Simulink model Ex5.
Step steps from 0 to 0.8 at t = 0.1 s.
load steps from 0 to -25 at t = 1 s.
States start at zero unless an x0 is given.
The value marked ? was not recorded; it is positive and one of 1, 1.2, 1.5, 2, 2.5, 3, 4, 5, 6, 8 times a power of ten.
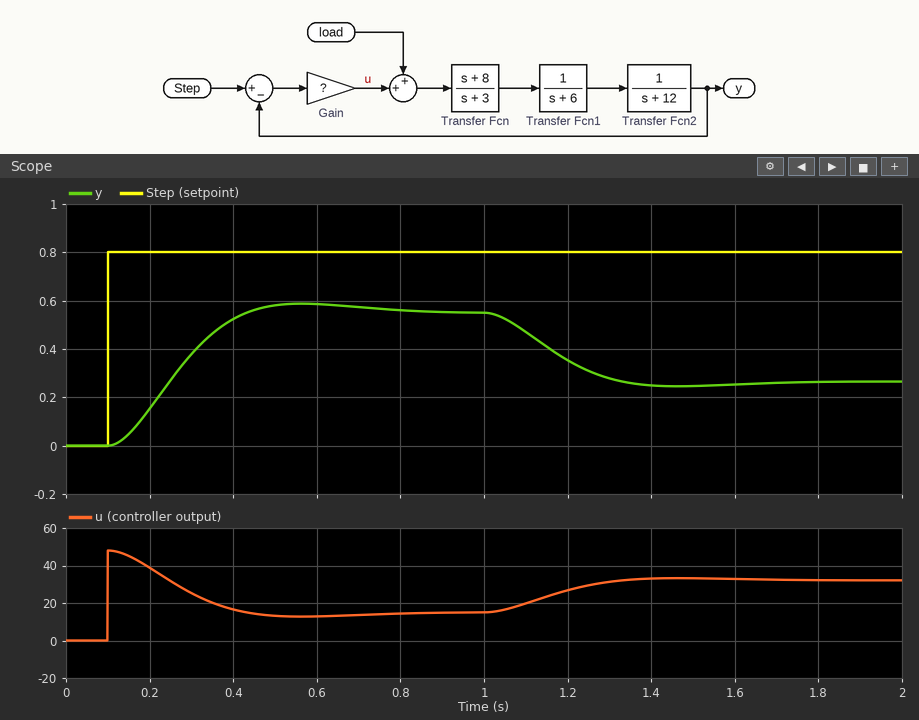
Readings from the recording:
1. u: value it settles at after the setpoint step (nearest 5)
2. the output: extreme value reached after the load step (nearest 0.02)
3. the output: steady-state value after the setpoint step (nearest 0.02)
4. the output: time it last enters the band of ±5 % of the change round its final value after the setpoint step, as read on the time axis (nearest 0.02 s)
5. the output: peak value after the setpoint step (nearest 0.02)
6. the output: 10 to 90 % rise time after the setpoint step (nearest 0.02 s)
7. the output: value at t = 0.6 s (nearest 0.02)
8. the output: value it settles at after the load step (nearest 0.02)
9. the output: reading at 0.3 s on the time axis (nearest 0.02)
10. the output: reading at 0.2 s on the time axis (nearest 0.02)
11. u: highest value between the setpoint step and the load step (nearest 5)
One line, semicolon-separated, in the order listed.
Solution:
15; 0.24; 0.56; 0.66 s; 0.58; 0.22 s; 0.58; 0.26; 0.38; 0.16; 50
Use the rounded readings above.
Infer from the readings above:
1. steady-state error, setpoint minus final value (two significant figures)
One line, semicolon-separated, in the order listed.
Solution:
0.24
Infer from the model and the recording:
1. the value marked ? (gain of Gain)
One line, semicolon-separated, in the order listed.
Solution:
60
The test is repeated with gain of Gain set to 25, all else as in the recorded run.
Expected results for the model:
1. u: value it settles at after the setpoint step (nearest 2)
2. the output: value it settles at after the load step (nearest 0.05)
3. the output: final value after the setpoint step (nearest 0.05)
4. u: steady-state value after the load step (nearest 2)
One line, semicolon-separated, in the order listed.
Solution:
10; -0.10; 0.40; 22
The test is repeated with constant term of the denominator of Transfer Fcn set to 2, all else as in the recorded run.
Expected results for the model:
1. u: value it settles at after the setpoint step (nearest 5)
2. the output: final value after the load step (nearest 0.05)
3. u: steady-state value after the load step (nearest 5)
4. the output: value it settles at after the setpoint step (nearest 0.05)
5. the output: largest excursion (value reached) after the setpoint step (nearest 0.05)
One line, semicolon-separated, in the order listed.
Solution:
10; 0.30; 30; 0.60; 0.65
